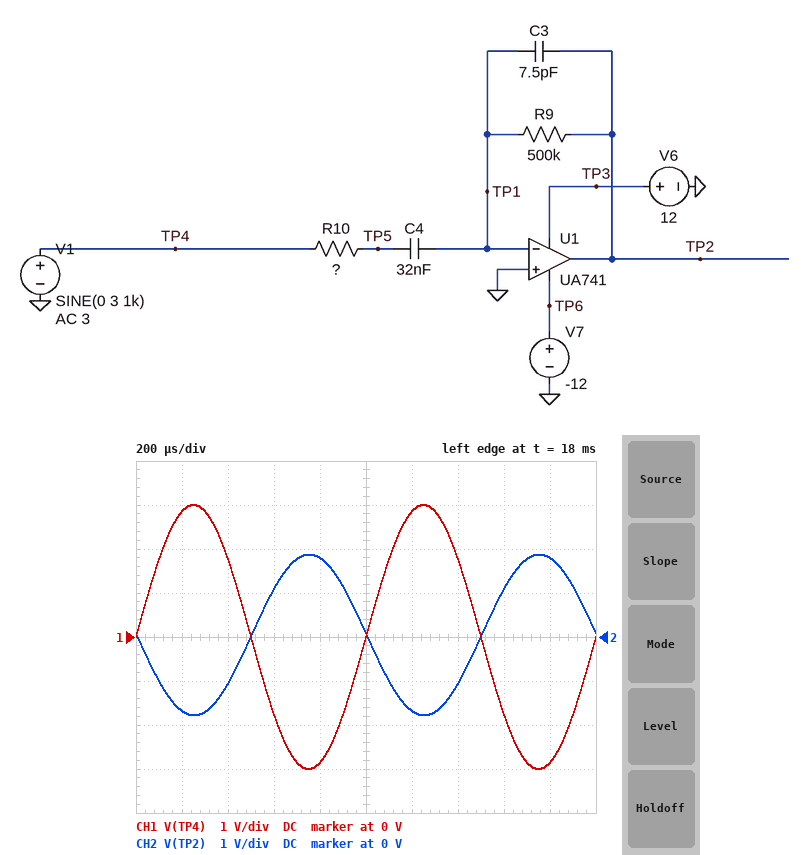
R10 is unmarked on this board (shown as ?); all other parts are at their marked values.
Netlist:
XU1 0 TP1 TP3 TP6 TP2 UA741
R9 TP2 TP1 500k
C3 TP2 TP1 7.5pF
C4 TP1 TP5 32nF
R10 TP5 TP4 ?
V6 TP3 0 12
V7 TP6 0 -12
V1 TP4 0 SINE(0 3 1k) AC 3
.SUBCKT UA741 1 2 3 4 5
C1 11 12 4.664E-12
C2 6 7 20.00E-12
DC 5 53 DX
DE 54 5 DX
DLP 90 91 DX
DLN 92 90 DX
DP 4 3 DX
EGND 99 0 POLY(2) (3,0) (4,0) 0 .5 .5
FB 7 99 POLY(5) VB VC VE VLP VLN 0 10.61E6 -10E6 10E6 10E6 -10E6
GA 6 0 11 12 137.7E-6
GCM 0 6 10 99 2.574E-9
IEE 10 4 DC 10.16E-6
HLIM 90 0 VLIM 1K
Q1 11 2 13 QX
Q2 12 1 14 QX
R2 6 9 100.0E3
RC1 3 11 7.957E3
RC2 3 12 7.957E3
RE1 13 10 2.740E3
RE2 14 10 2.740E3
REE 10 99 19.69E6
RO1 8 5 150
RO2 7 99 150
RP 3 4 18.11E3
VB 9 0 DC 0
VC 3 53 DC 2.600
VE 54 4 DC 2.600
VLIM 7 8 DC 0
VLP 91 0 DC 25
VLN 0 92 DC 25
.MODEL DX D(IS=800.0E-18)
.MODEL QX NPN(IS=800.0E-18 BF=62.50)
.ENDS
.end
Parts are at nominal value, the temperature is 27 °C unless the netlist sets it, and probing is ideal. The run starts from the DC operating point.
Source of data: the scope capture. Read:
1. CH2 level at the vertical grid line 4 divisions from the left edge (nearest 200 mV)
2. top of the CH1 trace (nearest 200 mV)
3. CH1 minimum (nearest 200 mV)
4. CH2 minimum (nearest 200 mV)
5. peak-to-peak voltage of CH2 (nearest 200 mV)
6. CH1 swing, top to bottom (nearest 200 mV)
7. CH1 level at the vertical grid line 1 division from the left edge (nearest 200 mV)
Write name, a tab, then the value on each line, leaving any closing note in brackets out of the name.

CH2 level at the vertical grid line 4 divisions from the left edge	1.8 V
top of the CH1 trace	3.0 V
CH1 minimum	-3.0 V
CH2 minimum	-1.8 V
peak-to-peak voltage of CH2	3.6 V
CH1 swing, top to bottom	6.0 V
CH1 level at the vertical grid line 1 division from the left edge	2.8 V
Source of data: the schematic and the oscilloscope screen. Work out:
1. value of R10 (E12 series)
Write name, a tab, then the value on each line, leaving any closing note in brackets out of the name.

value of R10	820 kΩ
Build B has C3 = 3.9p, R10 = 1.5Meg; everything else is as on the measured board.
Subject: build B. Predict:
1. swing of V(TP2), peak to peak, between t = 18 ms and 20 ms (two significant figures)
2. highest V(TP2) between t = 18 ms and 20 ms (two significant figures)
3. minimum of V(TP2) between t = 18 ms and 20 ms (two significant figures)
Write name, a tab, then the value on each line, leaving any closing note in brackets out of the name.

swing of V(TP2), peak to peak, between t = 18 ms and 20 ms	2.0 V
highest V(TP2) between t = 18 ms and 20 ms	1.0 V
minimum of V(TP2) between t = 18 ms and 20 ms	-960 mV
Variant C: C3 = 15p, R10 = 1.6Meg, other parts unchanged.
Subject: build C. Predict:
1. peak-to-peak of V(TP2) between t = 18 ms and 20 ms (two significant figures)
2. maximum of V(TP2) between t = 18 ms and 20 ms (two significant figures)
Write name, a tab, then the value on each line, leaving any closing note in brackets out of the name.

peak-to-peak of V(TP2) between t = 18 ms and 20 ms	1.9 V
maximum of V(TP2) between t = 18 ms and 20 ms	980 mV
